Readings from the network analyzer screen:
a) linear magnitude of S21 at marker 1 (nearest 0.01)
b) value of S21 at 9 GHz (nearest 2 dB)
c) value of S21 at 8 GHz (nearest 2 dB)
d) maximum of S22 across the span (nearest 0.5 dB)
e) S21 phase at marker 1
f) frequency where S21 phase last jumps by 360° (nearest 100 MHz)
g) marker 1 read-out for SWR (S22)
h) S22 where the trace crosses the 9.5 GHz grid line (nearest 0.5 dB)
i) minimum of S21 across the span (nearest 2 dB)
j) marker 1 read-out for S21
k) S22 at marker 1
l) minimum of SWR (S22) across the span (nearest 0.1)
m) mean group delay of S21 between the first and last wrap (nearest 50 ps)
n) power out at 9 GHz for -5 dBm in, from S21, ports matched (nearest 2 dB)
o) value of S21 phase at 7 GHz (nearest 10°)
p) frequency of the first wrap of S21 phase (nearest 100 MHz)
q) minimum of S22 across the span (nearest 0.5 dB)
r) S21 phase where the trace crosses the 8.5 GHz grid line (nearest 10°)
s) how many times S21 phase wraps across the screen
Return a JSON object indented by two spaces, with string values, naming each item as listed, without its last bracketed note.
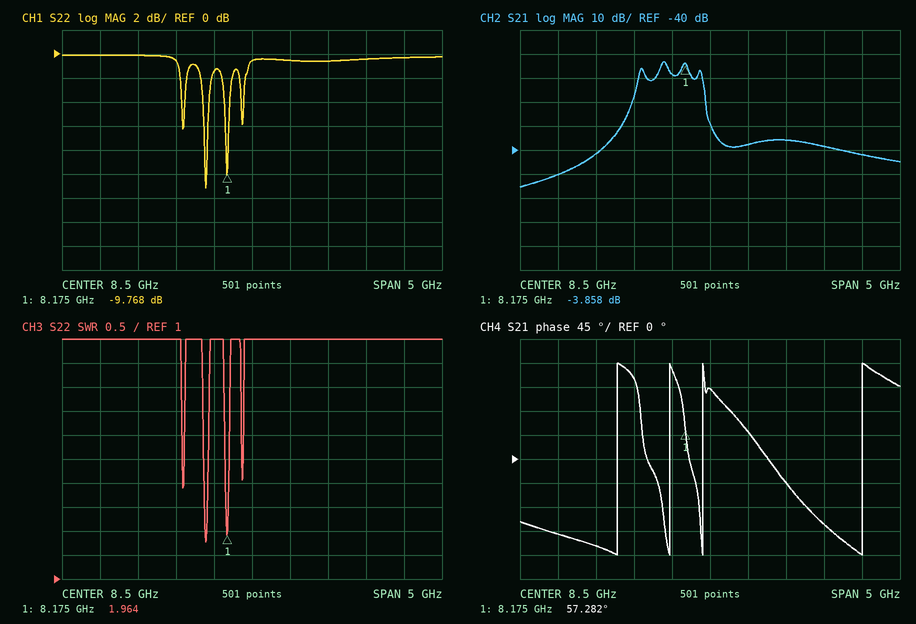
{
  "linear magnitude of S21 at marker 1": "0.64",
  "value of S21 at 9 GHz": "-38 dB",
  "value of S21 at 8 GHz": "-8 dB",
  "maximum of S22 across the span": "0.0 dB",
  "S21 phase at marker 1": "57.282°",
  "frequency where S21 phase last jumps by 360°": "10.5 GHz",
  "marker 1 read-out for SWR": "1.964",
  "S22 where the trace crosses the 9.5 GHz grid line": "-0.5 dB",
  "minimum of S21 across the span": "-56 dB",
  "marker 1 read-out for S21": "-3.858 dB",
  "S22 at marker 1": "-9.768 dB",
  "minimum of SWR (S22) across the span": "1.8",
  "mean group delay of S21 between the first and last wrap": "950 ps",
  "power out at 9 GHz for -5 dBm in, from S21, ports matched": "-42 dBm",
  "value of S21 phase at 7 GHz": "-160°",
  "frequency of the first wrap of S21 phase": "7.3 GHz",
  "minimum of S22 across the span": "-11.0 dB",
  "S21 phase where the trace crosses the 8.5 GHz grid line": "130°",
  "how many times S21 phase wraps across the screen": "4"
}
